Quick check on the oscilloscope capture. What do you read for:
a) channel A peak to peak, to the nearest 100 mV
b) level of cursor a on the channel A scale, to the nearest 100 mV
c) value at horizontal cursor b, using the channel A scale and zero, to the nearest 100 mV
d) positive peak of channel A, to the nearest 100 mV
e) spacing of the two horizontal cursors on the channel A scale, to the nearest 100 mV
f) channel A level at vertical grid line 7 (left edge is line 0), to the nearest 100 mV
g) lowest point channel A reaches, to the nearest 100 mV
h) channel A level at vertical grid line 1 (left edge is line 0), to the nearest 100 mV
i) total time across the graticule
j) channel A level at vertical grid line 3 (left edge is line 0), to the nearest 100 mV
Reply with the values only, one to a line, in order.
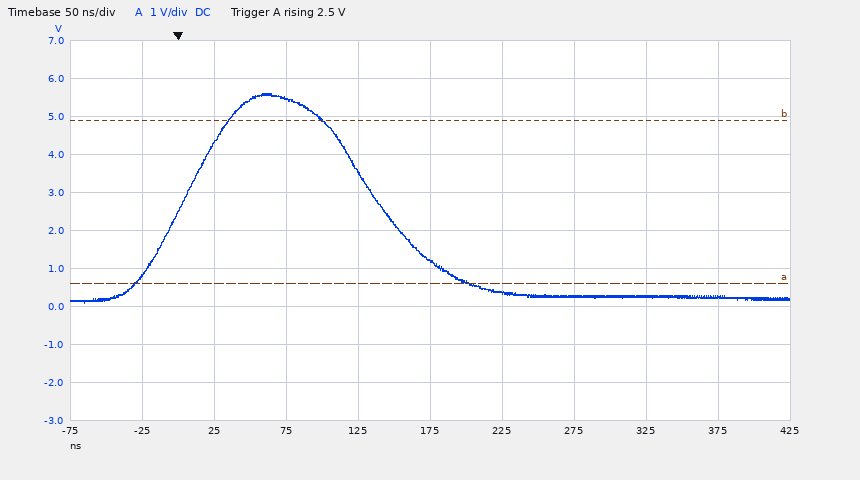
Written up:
5.5 V
600 mV
4.9 V
5.6 V
4.3 V
300 mV
100 mV
800 mV
500 ns
5.5 V
